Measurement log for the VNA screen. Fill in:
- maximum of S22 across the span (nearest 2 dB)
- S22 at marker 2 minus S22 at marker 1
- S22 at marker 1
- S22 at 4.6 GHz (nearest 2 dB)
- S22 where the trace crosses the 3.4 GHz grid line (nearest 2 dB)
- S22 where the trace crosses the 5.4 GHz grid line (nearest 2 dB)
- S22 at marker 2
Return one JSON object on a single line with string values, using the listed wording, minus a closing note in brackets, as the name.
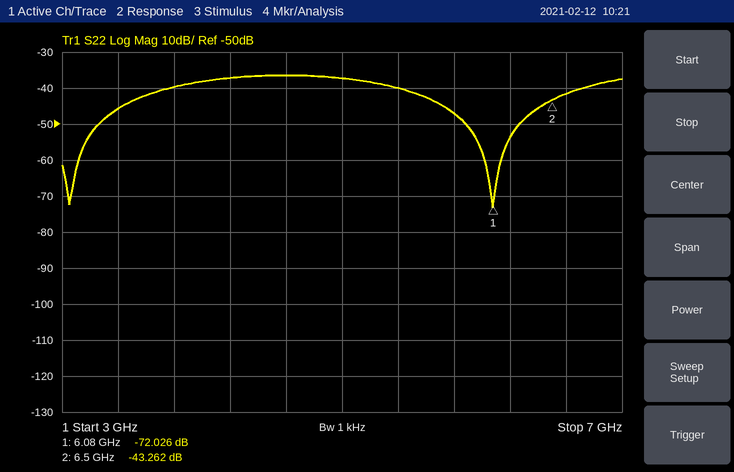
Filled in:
{"maximum of S22 across the span": "-36 dB", "S22 at marker 2 minus S22 at marker 1": "28.764 dB", "S22 at marker 1": "-72.026 dB", "S22 at 4.6 GHz": "-36 dB", "S22 where the trace crosses the 3.4 GHz grid line": "-46 dB", "S22 where the trace crosses the 5.4 GHz grid line": "-40 dB", "S22 at marker 2": "-43.262 dB"}
